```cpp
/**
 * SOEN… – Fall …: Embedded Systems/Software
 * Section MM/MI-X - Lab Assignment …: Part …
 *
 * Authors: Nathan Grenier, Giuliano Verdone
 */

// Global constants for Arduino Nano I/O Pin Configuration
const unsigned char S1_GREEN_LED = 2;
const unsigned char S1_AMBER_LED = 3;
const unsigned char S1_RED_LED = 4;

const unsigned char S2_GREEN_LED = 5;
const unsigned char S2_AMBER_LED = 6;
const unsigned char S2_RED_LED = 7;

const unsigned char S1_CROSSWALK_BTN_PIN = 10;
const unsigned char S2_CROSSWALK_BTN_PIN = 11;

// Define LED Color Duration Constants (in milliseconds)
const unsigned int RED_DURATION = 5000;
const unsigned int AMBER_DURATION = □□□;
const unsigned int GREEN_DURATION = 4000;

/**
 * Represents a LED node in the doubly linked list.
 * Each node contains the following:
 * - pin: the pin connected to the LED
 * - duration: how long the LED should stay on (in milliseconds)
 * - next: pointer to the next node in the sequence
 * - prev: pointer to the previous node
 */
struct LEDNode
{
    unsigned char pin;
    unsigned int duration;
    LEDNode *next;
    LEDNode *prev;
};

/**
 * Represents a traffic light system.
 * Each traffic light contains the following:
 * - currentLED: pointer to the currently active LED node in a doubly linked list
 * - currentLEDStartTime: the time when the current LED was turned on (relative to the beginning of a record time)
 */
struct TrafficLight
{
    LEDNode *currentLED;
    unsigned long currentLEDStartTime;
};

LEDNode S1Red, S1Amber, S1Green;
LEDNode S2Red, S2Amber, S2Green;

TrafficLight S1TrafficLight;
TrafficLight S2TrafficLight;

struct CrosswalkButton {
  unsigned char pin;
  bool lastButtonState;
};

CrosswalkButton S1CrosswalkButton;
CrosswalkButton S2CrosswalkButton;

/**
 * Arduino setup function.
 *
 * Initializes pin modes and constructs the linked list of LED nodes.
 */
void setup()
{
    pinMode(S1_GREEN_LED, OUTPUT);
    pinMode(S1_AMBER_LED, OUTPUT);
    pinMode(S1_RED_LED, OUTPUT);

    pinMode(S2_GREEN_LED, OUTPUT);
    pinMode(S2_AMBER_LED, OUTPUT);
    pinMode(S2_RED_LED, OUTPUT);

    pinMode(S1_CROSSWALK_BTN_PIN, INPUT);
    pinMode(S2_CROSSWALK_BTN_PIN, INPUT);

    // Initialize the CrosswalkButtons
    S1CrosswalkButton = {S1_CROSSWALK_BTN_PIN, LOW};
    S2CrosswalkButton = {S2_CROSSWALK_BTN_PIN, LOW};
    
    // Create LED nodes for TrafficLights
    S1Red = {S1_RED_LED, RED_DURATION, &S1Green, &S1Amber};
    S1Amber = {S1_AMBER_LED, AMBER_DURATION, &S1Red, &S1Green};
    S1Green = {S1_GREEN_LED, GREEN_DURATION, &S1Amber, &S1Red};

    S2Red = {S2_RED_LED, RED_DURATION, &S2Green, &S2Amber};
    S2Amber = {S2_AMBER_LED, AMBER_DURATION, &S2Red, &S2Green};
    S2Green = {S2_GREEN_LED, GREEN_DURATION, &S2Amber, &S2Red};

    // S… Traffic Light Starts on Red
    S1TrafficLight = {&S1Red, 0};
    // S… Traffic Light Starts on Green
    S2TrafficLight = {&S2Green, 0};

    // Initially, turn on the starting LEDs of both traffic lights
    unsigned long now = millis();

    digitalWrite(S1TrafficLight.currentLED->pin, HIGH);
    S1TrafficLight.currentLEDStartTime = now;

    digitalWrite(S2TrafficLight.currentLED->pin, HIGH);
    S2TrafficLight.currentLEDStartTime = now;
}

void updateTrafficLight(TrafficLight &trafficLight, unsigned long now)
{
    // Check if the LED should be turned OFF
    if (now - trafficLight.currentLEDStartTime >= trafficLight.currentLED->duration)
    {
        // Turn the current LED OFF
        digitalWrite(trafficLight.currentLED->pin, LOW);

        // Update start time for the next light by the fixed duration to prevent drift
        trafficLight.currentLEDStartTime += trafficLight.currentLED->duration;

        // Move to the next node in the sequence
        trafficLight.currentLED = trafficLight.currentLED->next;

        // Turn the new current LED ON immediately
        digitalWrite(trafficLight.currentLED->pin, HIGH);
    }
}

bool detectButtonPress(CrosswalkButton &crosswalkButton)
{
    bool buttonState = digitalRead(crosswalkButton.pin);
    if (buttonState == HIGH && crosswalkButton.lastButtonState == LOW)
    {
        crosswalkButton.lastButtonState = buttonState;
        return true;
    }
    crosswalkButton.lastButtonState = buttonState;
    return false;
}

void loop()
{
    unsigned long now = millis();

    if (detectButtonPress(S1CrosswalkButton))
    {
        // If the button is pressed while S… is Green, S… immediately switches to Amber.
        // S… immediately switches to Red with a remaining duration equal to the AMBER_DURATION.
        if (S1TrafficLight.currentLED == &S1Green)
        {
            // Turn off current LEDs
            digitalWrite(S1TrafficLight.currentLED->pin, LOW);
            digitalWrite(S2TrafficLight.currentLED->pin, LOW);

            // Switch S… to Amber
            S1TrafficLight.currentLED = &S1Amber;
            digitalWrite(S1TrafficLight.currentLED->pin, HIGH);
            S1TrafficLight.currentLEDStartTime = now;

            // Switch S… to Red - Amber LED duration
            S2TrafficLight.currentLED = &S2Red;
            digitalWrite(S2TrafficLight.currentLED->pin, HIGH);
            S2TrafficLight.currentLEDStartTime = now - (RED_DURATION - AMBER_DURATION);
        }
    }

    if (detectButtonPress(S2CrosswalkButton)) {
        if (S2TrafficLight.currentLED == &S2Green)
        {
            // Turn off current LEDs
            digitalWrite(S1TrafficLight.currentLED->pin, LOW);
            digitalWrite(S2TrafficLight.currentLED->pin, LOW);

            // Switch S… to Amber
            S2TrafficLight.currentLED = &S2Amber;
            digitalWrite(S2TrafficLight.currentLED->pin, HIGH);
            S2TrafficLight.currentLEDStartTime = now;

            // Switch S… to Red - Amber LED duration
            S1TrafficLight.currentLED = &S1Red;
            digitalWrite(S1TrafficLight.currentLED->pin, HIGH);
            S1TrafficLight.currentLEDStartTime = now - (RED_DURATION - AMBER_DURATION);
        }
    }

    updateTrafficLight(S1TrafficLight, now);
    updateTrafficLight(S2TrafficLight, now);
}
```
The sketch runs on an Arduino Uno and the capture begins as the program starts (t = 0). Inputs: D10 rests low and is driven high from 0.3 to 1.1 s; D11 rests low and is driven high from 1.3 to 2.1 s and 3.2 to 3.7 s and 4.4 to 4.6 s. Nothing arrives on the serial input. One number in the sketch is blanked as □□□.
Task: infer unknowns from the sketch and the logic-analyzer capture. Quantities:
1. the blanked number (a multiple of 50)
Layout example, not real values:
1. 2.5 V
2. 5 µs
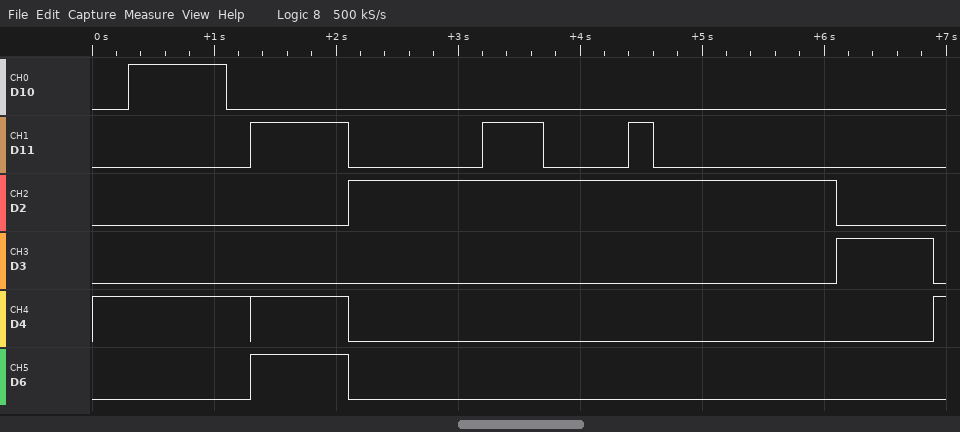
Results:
1. 800
